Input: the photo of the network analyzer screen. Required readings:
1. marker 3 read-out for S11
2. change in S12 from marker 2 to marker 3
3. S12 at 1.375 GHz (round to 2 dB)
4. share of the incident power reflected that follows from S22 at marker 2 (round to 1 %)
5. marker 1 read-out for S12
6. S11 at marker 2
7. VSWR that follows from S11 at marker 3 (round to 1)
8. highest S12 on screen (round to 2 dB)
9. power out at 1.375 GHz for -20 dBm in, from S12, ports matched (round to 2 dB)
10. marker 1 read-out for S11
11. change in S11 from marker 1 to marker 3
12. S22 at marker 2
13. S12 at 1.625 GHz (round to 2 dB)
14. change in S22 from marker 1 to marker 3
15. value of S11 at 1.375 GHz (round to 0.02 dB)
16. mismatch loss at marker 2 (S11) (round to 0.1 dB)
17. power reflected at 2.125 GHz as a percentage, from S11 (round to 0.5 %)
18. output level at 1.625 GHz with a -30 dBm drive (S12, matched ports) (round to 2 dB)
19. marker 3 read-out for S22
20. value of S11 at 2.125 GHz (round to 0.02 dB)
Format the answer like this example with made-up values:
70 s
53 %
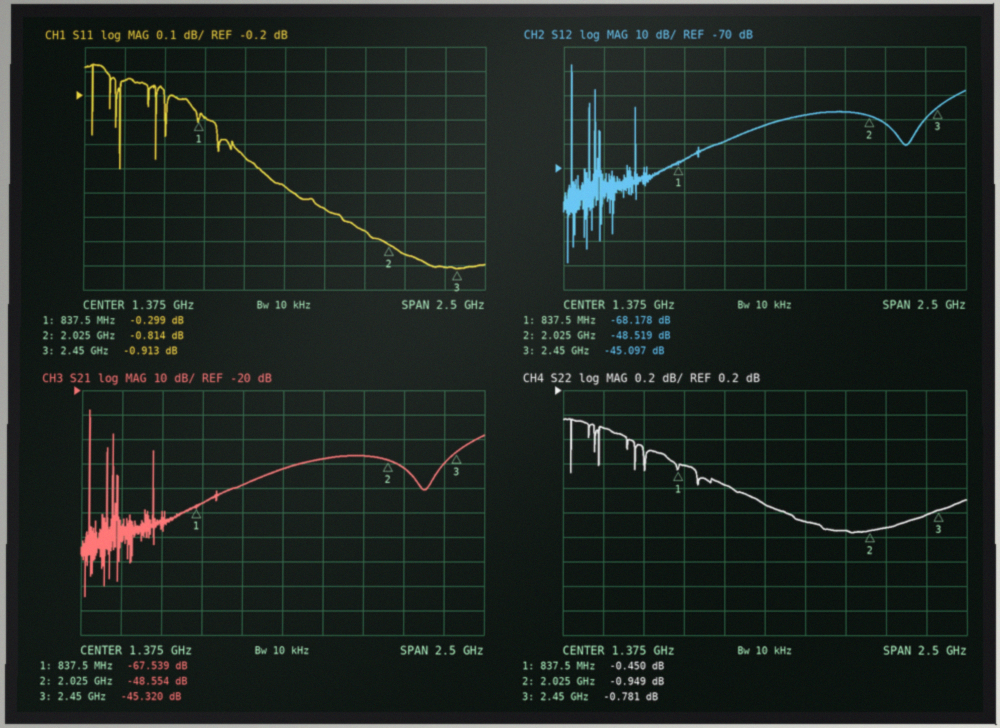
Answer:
-0.913 dB
3.422 dB
-52 dB
80 %
-68.178 dB
-0.814 dB
19
-28 dB
-72 dBm
-0.299 dB
-0.614 dB
-0.949 dB
-48 dB
-0.331 dB
-0.58 dB
7.7 dB
82.0 %
-78 dBm
-0.781 dB
-0.86 dB
